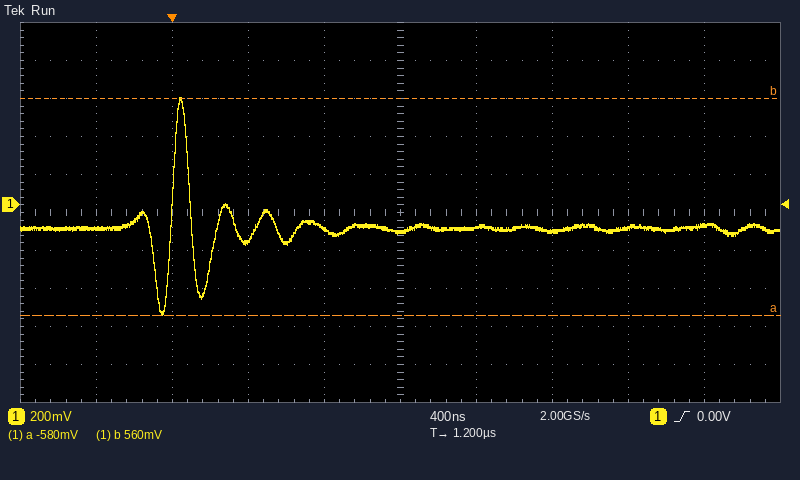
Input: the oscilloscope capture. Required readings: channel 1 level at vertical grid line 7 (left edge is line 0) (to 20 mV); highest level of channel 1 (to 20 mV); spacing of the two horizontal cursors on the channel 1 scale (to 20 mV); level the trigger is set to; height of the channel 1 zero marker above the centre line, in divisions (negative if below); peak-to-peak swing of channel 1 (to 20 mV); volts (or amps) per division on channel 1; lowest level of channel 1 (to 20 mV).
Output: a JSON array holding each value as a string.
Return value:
["-140 mV", "560 mV", "1.14 V", "0.00 V", "+0.2 div", "1.14 V", "200 mV", "-580 mV"]
